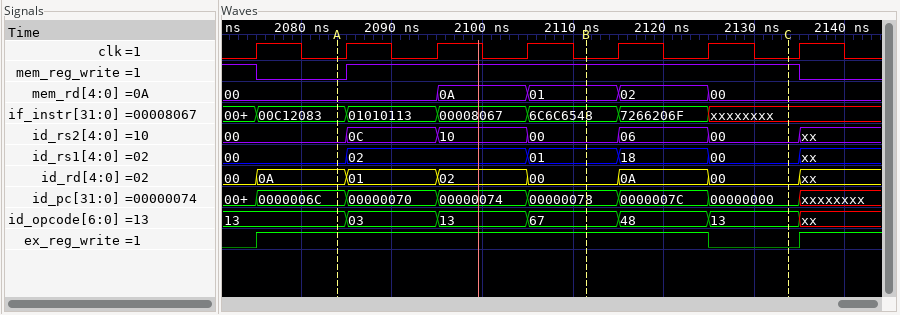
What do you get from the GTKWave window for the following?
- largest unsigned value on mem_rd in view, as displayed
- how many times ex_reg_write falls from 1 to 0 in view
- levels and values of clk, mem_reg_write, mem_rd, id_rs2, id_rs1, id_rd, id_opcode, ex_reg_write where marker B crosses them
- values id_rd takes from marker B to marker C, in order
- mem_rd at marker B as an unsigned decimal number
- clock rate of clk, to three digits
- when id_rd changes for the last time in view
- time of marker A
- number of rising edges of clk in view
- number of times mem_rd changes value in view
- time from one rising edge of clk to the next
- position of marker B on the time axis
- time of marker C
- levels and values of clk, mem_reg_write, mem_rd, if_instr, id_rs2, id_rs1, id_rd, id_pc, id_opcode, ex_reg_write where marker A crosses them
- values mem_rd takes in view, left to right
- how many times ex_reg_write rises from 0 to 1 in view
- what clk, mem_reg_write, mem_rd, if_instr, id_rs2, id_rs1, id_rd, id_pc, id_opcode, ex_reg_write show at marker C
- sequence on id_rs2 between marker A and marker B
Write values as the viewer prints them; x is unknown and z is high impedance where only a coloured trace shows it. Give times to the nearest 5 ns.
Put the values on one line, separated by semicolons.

0A; 1; clk=0, mem_reg_write=1, mem_rd=01, id_rs2=00, id_rs1=01, id_rd=00, id_opcode=67, ex_reg_write=1; 00, 0A, 00; 1; 100 MHz; 2135 ns; 2085 ns; 7; 4; 10 ns; 2110 ns; 2135 ns; clk=0, mem_reg_write=0, mem_rd=00, if_instr=00C12083, id_rs2=00, id_rs1=00, id_rd=0A, id_pc=0000006C, id_opcode=13, ex_reg_write=1; 00, 0A, 01, 02, 00; 2; clk=0, mem_reg_write=1, mem_rd=00, if_instr=xxxxxxxx, id_rs2=00, id_rs1=00, id_rd=00, id_pc=00000000, id_opcode=13, ex_reg_write=0; 00, 0C, 10, 00
